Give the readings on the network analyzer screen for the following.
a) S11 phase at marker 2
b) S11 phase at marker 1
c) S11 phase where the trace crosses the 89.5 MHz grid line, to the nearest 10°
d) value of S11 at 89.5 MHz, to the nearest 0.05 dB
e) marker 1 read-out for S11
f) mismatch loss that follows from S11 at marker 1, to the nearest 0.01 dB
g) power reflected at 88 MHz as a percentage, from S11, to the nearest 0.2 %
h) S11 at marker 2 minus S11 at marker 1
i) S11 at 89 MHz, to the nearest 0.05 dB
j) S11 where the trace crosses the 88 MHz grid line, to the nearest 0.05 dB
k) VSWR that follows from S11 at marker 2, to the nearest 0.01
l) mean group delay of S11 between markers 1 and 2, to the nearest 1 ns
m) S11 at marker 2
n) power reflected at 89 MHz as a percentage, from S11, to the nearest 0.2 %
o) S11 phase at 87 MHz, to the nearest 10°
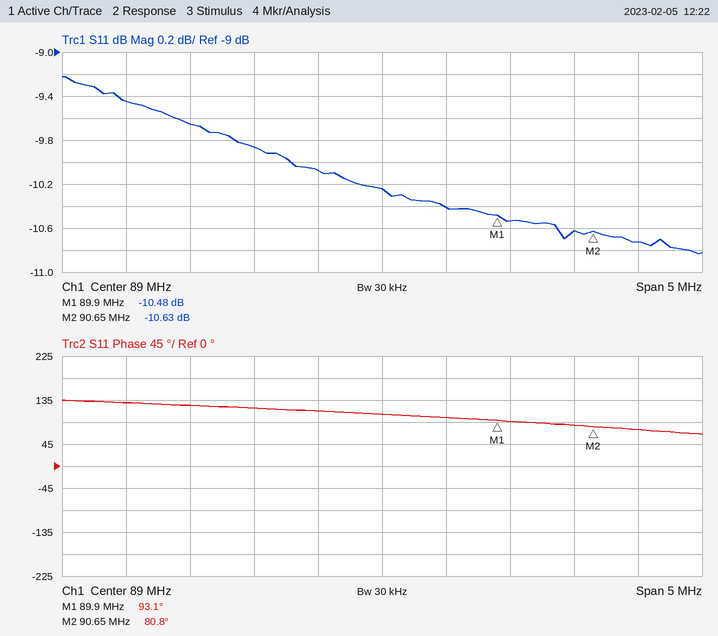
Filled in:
80.8°
93.1°
100°
-10.40 dB
-10.48 dB
0.41 dB
10.4 %
-0.15 dB
-10.25 dB
-9.85 dB
1.83
46 ns
-10.63 dB
9.4 %
130°
